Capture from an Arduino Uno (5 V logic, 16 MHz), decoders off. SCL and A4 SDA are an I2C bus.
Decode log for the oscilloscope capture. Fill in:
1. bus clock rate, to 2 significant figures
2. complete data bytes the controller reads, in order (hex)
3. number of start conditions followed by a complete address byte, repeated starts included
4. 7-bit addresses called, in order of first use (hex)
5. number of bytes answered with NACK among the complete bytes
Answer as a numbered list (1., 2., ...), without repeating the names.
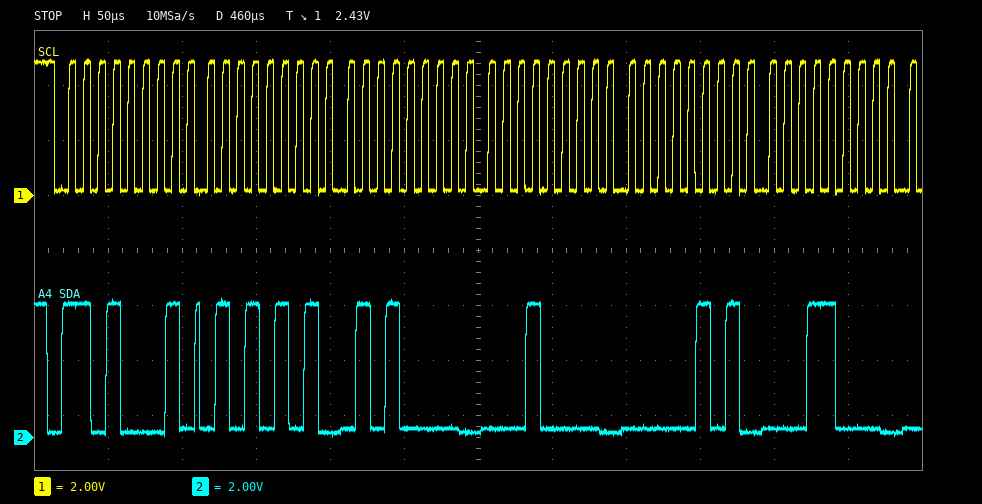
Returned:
1. 100 kHz
2. 55 50 10 05 18
3. 1
4. 0x68
5. 0
